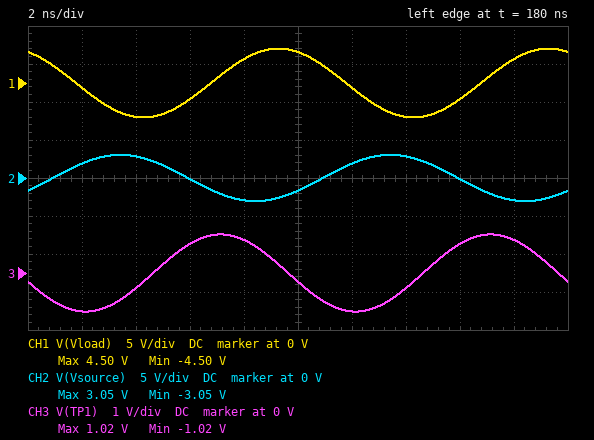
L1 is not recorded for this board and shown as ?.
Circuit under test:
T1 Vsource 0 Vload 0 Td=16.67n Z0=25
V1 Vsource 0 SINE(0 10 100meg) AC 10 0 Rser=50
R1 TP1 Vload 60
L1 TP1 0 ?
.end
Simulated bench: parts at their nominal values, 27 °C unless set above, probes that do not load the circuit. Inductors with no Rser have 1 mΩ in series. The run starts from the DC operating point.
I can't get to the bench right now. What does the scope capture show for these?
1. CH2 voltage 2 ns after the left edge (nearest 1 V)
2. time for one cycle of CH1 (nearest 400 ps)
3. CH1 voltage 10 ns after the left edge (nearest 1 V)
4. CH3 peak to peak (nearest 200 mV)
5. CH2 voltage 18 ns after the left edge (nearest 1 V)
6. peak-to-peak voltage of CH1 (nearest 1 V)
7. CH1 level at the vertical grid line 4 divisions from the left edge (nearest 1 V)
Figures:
2 V
10.0 ns
4 V
2.0 V
-3 V
9 V
3 V
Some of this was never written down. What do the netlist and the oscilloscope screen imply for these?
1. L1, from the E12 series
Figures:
22 nH
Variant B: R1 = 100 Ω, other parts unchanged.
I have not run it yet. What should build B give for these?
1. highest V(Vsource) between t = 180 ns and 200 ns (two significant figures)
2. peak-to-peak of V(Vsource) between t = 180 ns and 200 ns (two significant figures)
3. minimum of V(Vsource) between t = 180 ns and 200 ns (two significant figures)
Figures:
2.8 V
5.5 V
-2.8 V
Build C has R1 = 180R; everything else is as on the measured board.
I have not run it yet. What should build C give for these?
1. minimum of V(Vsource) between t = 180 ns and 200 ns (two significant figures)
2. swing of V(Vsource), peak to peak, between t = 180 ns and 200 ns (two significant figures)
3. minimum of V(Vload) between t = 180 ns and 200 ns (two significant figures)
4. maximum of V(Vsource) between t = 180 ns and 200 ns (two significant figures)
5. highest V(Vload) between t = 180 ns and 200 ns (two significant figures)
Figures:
-2.7 V
5.3 V
-5.1 V
2.7 V
5.1 V
